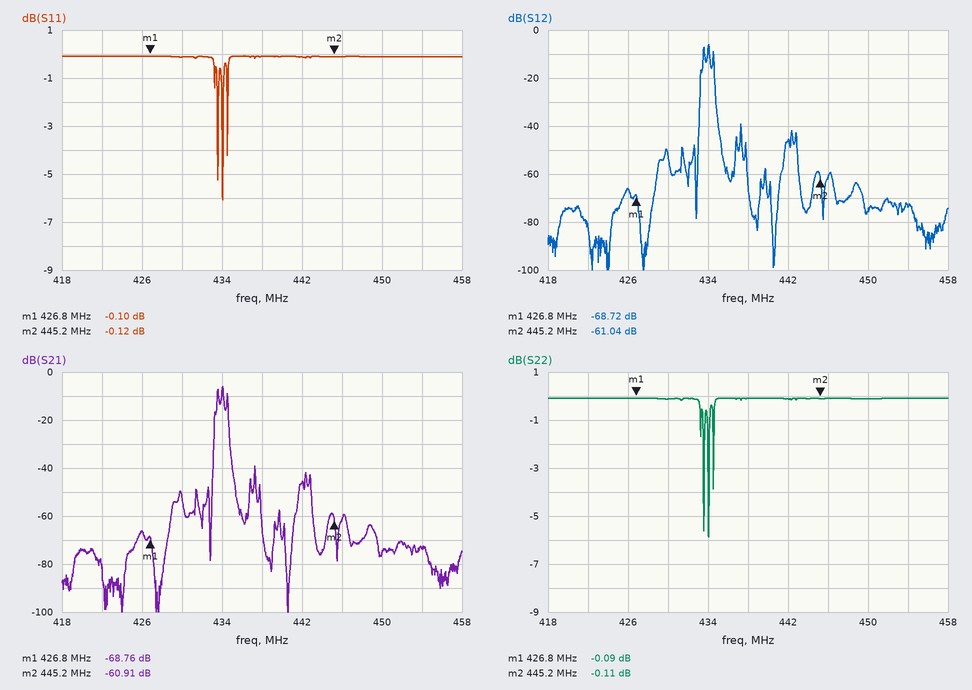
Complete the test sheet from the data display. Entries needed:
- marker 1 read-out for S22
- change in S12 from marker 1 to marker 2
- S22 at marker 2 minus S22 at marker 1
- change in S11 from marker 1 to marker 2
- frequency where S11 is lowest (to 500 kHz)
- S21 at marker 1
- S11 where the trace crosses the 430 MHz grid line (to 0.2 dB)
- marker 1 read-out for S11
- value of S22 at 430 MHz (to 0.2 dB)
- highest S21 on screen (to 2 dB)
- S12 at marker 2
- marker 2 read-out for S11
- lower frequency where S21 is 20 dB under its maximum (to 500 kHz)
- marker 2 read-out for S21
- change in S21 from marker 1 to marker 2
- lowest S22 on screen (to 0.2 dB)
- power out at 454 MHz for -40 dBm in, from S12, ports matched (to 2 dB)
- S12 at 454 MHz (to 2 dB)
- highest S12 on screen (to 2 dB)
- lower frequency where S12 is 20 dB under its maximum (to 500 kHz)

-0.09 dB
7.68 dB
-0.02 dB
-0.02 dB
434.0 MHz
-68.76 dB
-0.2 dB
-0.10 dB
-0.2 dB
-6 dB
-61.04 dB
-0.12 dB
433.0 MHz
-60.91 dB
7.85 dB
-5.8 dB
-114 dBm
-74 dB
-6 dB
433.0 MHz
